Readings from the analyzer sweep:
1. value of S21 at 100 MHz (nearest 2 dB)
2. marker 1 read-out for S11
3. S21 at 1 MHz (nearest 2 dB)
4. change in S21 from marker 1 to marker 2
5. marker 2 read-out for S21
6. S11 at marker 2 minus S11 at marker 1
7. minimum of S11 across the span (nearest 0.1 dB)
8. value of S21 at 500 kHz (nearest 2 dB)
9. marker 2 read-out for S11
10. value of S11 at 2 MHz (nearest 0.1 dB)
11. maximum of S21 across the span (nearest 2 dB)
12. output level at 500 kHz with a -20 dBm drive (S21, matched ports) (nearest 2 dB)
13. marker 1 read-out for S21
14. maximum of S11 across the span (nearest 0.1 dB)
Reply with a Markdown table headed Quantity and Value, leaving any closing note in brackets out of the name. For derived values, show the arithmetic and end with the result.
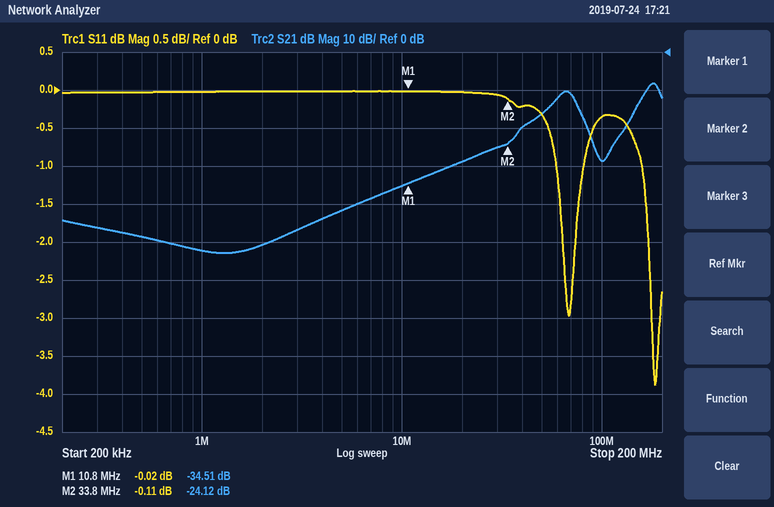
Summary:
| Quantity | Value |
|---|---|
| value of S21 at 100 MHz | -28 dB |
| marker 1 read-out for S11 | -0.02 dB |
| S21 at 1 MHz | -52 dB |
| change in S21 from marker 1 to marker 2 | -24.12 − (-34.51) = 10.39 dB |
| marker 2 read-out for S21 | -24.12 dB |
| S11 at marker 2 minus S11 at marker 1 | -0.11 − (-0.02) = -0.09 dB |
| minimum of S11 across the span | -3.9 dB |
| value of S21 at 500 kHz | -48 dB |
| marker 2 read-out for S11 | -0.11 dB |
| value of S11 at 2 MHz | 0.0 dB |
| maximum of S21 across the span | -8 dB |
| output level at 500 kHz with a -20 dBm drive (S21, matched ports) | -20 dBm + (-48 dB) = -68 dBm |
| marker 1 read-out for S21 | -34.51 dB |
| maximum of S11 across the span | 0.0 dB |
